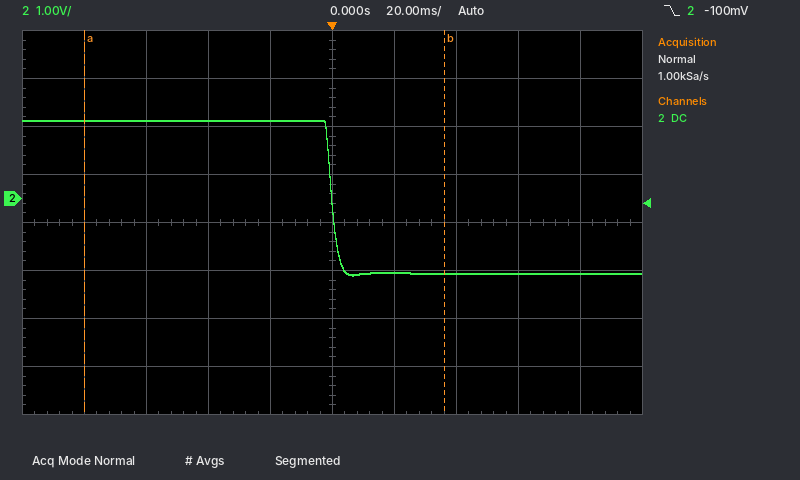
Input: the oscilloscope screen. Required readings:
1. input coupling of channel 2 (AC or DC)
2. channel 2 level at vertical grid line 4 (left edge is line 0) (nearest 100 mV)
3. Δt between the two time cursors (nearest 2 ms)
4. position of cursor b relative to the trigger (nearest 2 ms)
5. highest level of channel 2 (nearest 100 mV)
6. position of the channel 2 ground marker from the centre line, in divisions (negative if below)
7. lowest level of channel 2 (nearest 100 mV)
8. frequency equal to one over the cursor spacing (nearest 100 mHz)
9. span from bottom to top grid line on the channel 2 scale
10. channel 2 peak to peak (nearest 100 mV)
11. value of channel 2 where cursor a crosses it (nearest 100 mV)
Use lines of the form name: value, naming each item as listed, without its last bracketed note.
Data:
input coupling of channel 2: DC
channel 2 level at vertical grid line 4 (left edge is line 0): 1.6 V
Δt between the two time cursors: 116 ms
position of cursor b relative to the trigger: +36 ms
highest level of channel 2: 1.6 V
position of the channel 2 ground marker from the centre line, in divisions: +0.5 div
lowest level of channel 2: -1.6 V
frequency equal to one over the cursor spacing: 8.6 Hz
span from bottom to top grid line on the channel 2 scale: 8 V
channel 2 peak to peak: 3.2 V
value of channel 2 where cursor a crosses it: 1.6 V
